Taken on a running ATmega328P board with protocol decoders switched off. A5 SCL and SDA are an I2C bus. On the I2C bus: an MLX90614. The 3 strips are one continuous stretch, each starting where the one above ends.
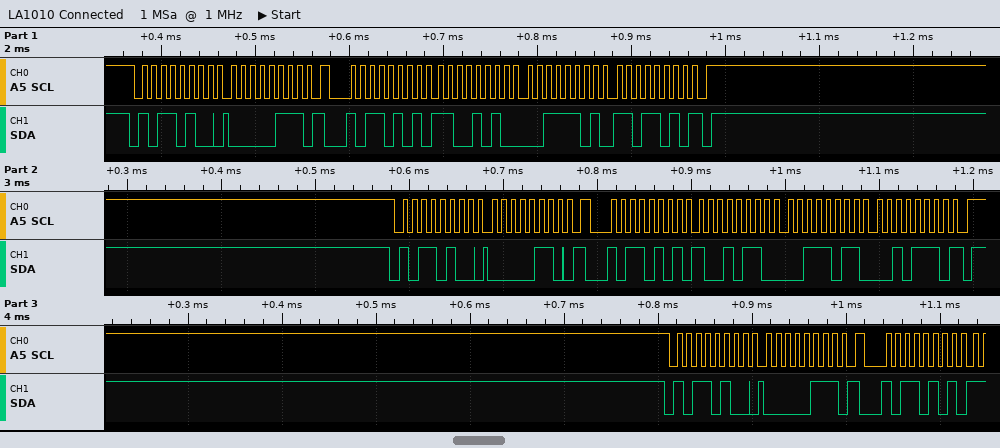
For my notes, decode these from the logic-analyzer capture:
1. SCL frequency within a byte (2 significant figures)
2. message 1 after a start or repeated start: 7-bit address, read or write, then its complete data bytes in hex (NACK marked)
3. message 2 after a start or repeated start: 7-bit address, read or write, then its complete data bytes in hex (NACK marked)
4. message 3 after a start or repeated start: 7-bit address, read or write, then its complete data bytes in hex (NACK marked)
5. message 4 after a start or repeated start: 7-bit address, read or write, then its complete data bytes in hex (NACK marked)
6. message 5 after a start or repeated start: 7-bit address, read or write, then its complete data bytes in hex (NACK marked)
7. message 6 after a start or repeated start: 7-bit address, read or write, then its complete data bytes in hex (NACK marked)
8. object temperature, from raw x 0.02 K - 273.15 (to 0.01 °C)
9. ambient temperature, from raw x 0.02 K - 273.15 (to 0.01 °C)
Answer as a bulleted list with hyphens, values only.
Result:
- 100 kHz
- 0x5A write: 07
- 0x5A read: CA 3D DA NACK
- 0x5A write: 06
- 0x5A read: 96 3B 2E NACK
- 0x5A write: 07
- 0x5A read
- 43.21 °C
- 31.93 °C
